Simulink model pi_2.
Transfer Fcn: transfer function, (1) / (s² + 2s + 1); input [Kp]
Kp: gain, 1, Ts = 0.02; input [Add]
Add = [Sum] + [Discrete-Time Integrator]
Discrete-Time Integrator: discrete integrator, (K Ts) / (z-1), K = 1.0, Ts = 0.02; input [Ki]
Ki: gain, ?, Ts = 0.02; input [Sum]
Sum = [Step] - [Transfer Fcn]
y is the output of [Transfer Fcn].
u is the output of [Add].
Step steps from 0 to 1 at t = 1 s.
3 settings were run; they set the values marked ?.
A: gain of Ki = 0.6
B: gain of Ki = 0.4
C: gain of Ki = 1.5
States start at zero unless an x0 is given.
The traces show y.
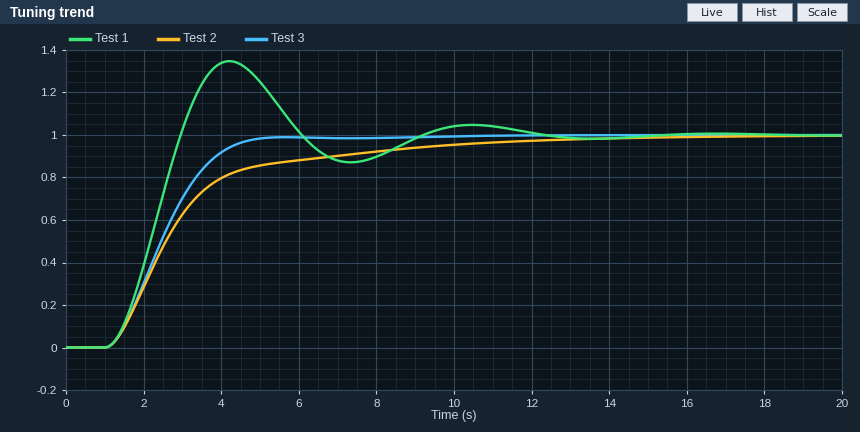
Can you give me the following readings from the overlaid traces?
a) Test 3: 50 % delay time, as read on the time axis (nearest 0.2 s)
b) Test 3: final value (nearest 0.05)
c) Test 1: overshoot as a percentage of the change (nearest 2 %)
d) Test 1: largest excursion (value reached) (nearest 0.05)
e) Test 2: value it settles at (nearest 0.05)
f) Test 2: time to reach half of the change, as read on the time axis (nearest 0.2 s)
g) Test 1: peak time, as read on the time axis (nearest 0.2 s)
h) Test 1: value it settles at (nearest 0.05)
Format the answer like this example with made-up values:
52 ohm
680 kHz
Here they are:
2.4 s
1.00
34 %
1.35
1.00
2.6 s
4.2 s
1.00
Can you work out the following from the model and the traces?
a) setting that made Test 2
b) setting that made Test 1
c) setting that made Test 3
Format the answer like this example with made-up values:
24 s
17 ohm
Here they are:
B
C
A
